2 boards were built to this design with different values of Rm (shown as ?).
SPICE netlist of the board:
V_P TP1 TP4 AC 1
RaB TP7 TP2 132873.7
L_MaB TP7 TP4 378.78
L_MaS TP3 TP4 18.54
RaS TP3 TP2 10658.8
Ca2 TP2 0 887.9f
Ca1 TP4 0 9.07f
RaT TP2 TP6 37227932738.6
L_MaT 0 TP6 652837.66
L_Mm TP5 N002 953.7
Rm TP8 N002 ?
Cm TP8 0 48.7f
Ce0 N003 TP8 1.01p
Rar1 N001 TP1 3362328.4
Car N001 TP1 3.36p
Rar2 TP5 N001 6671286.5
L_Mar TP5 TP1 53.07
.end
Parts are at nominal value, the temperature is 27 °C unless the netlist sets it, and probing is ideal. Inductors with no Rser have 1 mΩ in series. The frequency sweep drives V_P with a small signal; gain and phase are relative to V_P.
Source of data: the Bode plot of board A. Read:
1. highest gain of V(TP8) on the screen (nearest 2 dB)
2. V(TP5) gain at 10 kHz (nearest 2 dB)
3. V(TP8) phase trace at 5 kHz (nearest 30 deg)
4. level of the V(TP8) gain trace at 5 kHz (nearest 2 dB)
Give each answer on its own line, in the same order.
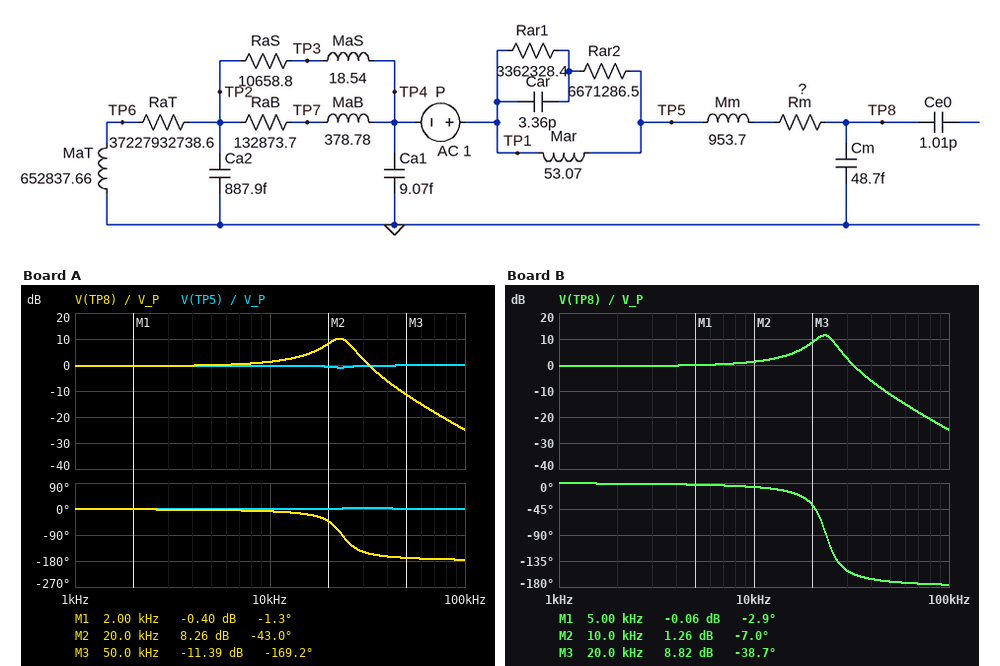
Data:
10 dB
0 dB
0 deg
0 dB
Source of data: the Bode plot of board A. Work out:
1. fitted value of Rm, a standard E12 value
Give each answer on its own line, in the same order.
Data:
39 MΩ
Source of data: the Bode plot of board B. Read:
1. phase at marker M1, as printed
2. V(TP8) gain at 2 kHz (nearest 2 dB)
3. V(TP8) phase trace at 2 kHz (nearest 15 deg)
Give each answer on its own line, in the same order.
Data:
-2.9 deg
0 dB
0 deg
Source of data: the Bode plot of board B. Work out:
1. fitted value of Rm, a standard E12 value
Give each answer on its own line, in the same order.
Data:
33 MΩ
